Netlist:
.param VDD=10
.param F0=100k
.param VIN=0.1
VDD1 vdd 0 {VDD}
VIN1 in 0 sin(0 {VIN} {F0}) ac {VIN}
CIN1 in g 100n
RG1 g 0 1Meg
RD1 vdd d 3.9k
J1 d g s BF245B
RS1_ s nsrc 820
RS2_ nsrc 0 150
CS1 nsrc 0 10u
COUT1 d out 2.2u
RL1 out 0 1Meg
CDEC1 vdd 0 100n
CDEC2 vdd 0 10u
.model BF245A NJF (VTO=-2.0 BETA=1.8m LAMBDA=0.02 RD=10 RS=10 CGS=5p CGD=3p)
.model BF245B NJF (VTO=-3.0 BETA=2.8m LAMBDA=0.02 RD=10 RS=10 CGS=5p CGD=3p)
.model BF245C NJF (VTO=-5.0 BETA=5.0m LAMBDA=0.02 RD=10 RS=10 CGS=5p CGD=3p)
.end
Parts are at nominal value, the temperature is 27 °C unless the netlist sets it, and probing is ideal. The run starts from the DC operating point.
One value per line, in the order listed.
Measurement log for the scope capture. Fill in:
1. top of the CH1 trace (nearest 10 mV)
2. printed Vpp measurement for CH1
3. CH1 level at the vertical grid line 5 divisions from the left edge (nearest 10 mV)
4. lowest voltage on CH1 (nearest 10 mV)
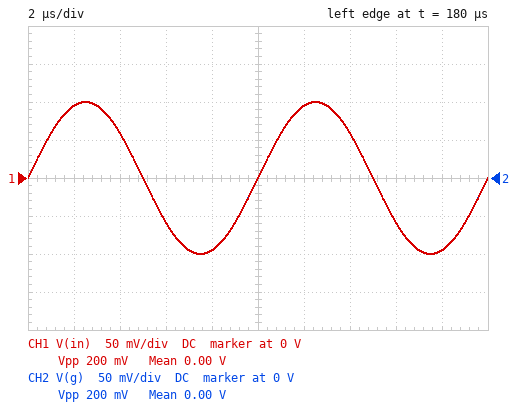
100 mV
200 mV
0 V
-100 mV
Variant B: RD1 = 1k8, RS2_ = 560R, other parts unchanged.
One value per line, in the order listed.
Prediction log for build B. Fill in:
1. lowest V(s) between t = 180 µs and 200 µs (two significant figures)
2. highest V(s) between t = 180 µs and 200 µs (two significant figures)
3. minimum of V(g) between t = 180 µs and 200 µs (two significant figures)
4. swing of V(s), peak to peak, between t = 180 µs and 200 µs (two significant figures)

2.2 V
2.3 V
-100 mV
150 mV
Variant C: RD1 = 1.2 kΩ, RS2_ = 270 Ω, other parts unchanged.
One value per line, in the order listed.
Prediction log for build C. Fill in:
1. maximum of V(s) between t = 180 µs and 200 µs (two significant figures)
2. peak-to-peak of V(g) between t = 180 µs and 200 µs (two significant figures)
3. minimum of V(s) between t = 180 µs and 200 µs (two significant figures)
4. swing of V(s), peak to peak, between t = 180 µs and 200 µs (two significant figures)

2.3 V
200 mV
2.1 V
160 mV
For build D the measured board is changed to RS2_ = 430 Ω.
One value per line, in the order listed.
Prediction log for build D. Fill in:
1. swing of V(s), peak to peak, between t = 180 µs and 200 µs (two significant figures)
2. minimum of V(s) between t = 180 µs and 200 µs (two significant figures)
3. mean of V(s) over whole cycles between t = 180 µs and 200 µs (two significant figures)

130 mV
2.1 V
2.2 V
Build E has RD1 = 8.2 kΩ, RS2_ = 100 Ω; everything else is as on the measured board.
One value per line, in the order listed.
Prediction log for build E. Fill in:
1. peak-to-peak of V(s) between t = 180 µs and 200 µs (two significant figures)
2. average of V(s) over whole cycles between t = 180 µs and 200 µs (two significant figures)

1.1 mV
1.0 V
